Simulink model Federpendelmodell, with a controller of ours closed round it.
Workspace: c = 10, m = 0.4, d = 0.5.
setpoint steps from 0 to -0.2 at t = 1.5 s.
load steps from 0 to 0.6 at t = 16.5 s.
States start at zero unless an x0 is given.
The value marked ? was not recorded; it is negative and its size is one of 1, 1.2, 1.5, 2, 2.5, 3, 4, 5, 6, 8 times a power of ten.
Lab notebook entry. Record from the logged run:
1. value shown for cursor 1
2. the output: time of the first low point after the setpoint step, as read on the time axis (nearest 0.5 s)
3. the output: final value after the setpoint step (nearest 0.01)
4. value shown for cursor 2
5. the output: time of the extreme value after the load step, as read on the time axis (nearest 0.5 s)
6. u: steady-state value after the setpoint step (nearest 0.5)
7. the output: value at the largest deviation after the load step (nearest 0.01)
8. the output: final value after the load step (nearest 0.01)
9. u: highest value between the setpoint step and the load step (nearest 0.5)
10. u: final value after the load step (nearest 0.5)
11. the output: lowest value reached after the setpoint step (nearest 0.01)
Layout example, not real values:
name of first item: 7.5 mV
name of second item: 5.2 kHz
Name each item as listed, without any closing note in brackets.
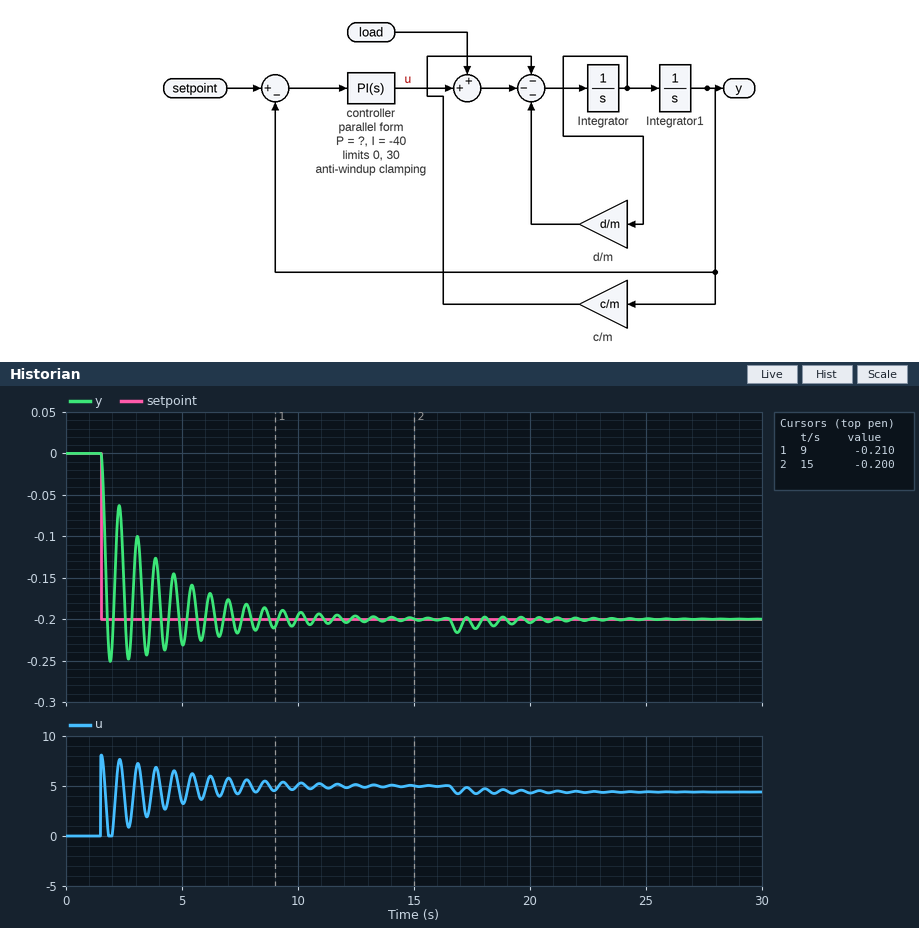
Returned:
value shown for cursor 1: -0.210
the output: time of the first low point after the setpoint step, as read on the time axis: 2.0 s
the output: final value after the setpoint step: -0.20
value shown for cursor 2: -0.200
the output: time of the extreme value after the load step, as read on the time axis: 17.0 s
u: steady-state value after the setpoint step: 5.0
the output: value at the largest deviation after the load step: -0.22
the output: final value after the load step: -0.20
u: highest value between the setpoint step and the load step: 8.0
u: final value after the load step: 4.5
the output: lowest value reached after the setpoint step: -0.25
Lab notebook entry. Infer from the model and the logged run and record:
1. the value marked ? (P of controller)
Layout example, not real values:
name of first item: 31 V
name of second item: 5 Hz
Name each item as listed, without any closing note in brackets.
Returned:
the value marked ?: -40
